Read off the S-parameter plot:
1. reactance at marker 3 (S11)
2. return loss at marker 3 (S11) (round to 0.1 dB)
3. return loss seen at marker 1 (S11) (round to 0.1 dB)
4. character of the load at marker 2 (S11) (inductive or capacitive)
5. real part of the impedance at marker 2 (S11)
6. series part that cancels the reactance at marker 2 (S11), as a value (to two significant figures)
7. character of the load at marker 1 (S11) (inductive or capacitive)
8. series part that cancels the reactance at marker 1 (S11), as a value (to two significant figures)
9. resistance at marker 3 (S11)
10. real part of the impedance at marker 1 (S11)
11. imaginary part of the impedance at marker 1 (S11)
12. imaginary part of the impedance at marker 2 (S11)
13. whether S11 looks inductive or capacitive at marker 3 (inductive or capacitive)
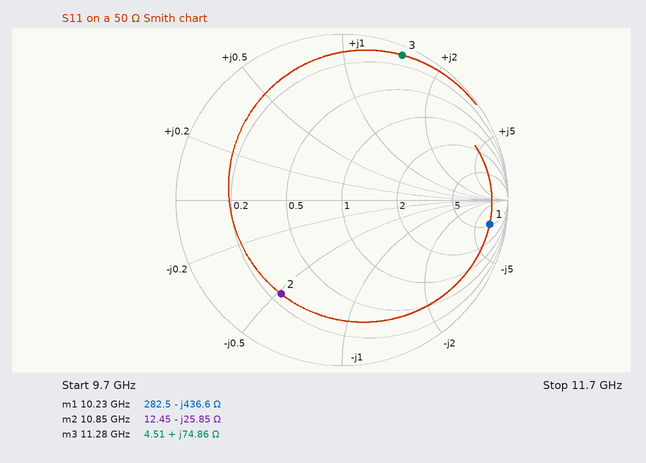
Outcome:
+74.86 Ω
0.5 dB
0.9 dB
capacitive
12.45 Ω
380 pH
capacitive
6.8 nH
4.51 Ω
282.5 Ω
-436.6 Ω
-25.85 Ω
inductive
